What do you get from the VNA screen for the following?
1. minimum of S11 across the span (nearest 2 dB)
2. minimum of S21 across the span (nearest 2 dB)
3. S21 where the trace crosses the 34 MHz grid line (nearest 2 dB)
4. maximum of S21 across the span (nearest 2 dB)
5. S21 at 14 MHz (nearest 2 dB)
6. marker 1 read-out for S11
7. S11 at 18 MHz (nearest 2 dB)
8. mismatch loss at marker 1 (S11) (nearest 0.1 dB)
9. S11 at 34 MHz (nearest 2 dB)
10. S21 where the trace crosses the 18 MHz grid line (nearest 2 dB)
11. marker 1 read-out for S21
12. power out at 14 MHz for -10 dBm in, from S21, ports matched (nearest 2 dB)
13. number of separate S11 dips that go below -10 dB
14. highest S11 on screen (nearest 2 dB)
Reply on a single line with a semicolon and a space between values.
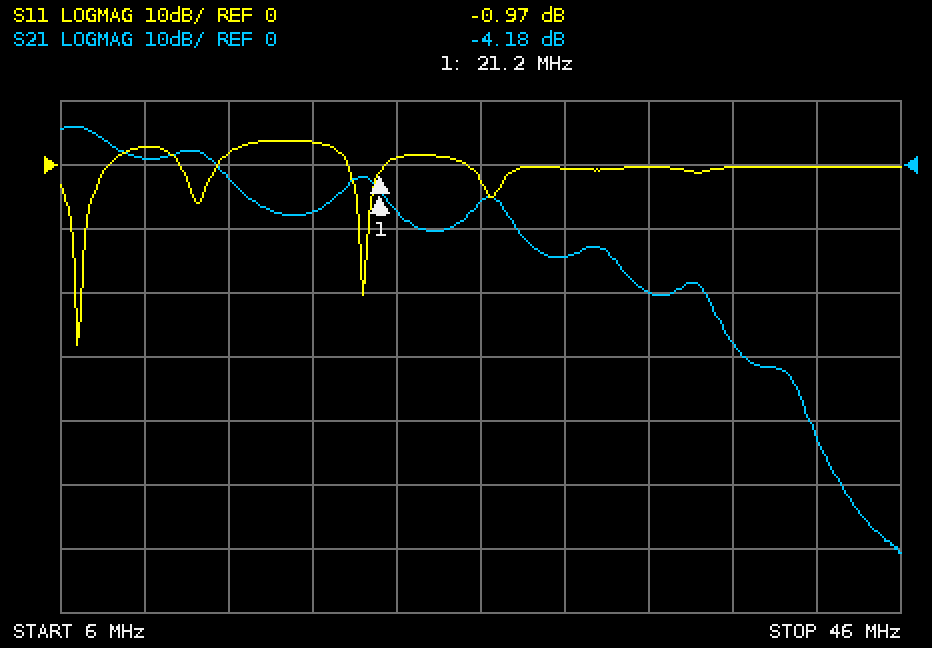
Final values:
-28 dB; -60 dB; -20 dB; 6 dB; -2 dB; -0.97 dB; 4 dB; 7.0 dB; 0 dB; -8 dB; -4.18 dB; -12 dBm; 2; 4 dB
